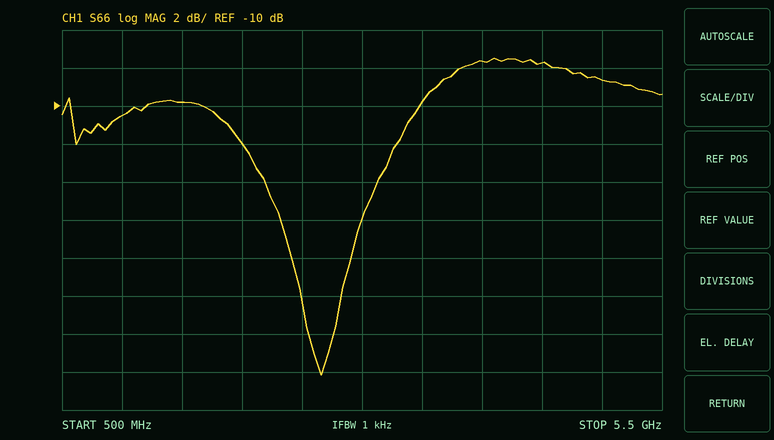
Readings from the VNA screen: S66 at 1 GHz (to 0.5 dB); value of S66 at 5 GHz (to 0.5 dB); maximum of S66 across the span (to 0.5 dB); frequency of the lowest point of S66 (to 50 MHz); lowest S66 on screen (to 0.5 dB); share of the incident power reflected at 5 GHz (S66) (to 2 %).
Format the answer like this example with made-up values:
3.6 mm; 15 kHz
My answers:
-10.5 dB; -8.5 dB; -7.5 dB; 2.65 GHz; -24.0 dB; 14 %
